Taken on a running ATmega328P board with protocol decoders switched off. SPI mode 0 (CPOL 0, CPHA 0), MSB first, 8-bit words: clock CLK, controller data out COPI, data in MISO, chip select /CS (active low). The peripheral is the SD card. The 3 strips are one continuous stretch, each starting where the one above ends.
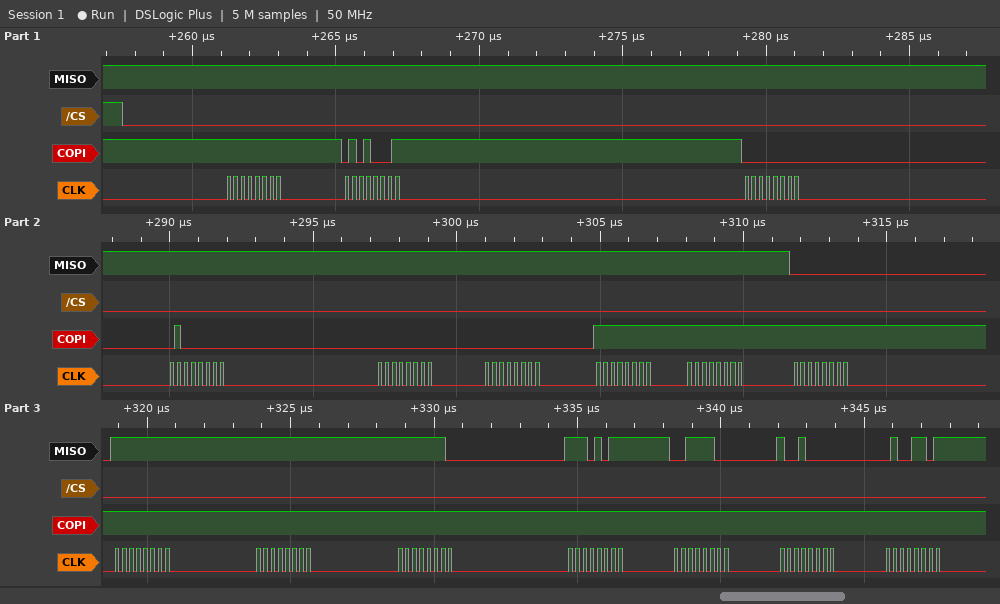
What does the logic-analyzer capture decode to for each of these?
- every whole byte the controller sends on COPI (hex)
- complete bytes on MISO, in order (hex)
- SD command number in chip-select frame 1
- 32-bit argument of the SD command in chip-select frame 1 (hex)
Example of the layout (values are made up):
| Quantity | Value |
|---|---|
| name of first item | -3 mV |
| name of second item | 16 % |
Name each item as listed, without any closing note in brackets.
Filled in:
| Quantity | Value |
|---|---|
| every whole byte the controller sends on COPI | 0xFF 0x51 0x00 0x40 0x00 0x00 0xFF 0xFF 0xFF 0xFF 0xFF 0xFF 0xFF 0xFF 0xFF 0xFF |
| complete bytes on MISO, in order | 0xFF 0xFF 0xFF 0xFF 0xFF 0xFF 0xFF 0xFF 0x00 0xFF 0xFF 0xFE 0xEB 0x3C 0x90 0x4D |
| SD command number in chip-select frame 1 | CMD17 |
| 32-bit argument of the SD command in chip-select frame 1 | 0x00400000 |
